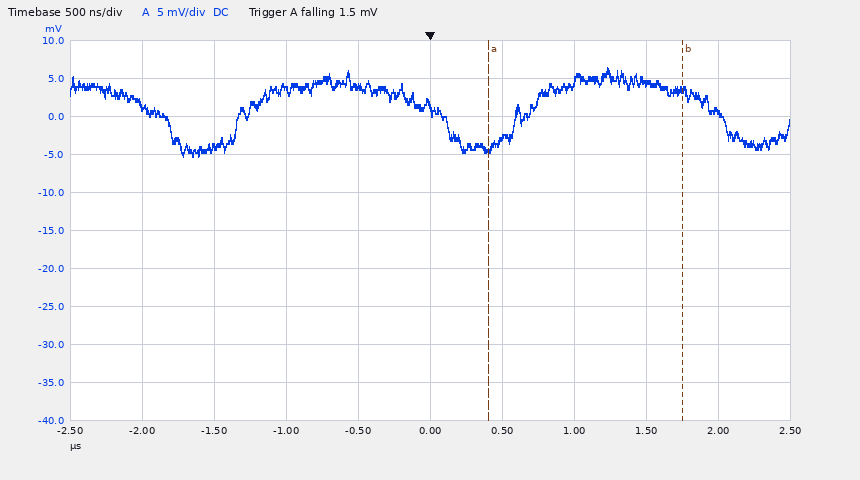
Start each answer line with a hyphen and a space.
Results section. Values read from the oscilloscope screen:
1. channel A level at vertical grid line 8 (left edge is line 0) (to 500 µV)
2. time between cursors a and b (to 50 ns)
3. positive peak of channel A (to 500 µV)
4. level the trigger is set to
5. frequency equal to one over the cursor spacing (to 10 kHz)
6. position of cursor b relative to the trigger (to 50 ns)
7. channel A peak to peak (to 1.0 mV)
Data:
- 4.5 mV
- 1.35 µs
- 6.5 mV
- 1.5 mV
- 740 kHz
- +1.75 µs
- 12.0 mV
